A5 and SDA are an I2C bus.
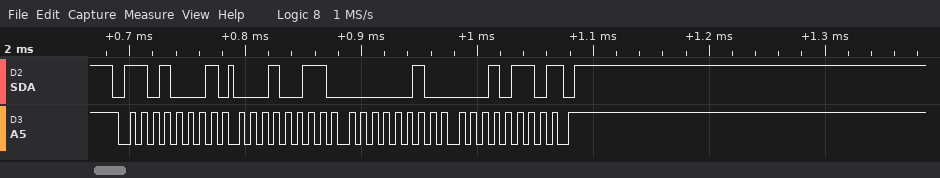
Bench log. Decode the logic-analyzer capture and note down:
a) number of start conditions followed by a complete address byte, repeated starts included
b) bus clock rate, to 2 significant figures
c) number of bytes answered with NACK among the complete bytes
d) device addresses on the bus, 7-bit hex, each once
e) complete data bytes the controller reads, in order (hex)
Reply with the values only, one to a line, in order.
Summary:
1
100 kHz
1
0x68
13 02 16
